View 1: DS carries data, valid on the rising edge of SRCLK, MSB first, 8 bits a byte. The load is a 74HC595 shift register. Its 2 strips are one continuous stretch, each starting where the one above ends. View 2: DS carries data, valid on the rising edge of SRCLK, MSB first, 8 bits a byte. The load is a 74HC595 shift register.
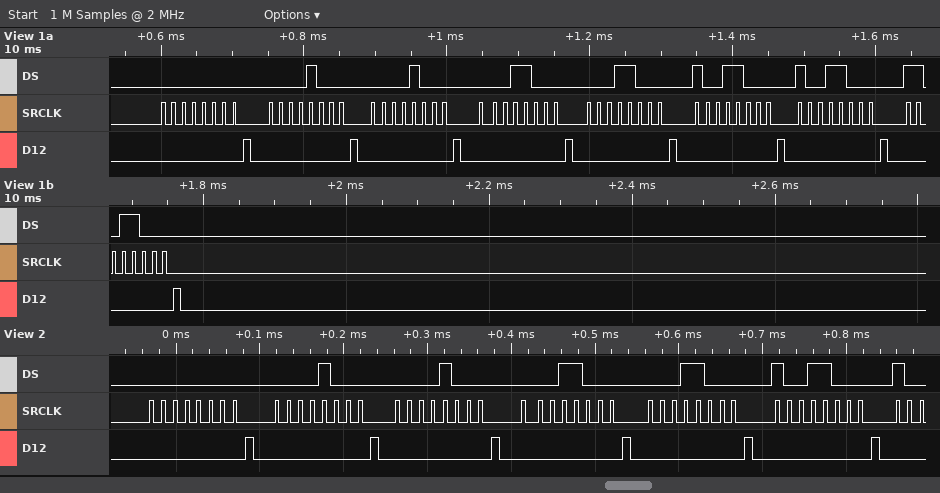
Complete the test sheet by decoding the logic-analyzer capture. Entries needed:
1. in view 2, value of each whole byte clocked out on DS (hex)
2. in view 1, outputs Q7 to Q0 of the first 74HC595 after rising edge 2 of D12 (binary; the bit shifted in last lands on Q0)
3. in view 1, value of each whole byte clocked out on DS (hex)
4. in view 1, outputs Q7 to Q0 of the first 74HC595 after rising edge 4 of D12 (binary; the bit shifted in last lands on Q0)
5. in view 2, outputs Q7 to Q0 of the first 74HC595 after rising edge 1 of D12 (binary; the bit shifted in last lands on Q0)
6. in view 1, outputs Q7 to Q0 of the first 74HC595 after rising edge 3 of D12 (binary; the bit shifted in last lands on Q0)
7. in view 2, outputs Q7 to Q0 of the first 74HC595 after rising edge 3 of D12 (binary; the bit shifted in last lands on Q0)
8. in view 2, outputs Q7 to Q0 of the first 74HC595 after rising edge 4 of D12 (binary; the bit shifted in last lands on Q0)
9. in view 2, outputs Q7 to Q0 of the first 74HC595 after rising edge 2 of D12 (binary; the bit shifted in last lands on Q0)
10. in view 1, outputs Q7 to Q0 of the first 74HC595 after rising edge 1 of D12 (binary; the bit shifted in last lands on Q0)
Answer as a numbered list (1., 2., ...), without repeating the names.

1. 00 08 08 18 18 98
2. 00001000
3. 00 08 08 18 18 98 98 D8
4. 00011000
5. 00000000
6. 00001000
7. 00001000
8. 00011000
9. 00001000
10. 00000000
